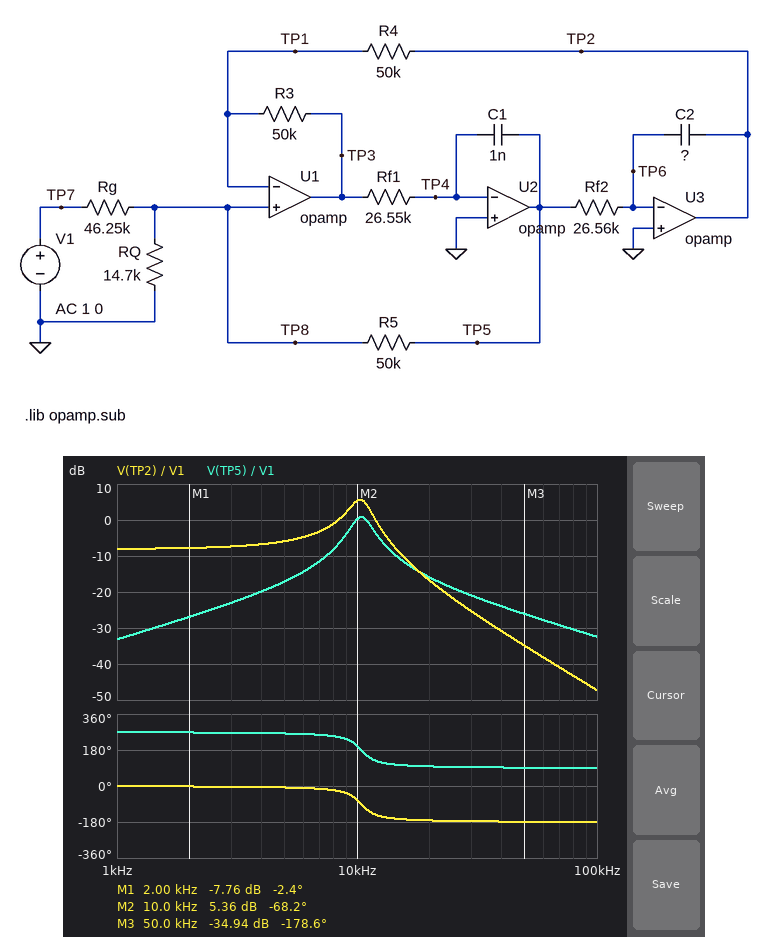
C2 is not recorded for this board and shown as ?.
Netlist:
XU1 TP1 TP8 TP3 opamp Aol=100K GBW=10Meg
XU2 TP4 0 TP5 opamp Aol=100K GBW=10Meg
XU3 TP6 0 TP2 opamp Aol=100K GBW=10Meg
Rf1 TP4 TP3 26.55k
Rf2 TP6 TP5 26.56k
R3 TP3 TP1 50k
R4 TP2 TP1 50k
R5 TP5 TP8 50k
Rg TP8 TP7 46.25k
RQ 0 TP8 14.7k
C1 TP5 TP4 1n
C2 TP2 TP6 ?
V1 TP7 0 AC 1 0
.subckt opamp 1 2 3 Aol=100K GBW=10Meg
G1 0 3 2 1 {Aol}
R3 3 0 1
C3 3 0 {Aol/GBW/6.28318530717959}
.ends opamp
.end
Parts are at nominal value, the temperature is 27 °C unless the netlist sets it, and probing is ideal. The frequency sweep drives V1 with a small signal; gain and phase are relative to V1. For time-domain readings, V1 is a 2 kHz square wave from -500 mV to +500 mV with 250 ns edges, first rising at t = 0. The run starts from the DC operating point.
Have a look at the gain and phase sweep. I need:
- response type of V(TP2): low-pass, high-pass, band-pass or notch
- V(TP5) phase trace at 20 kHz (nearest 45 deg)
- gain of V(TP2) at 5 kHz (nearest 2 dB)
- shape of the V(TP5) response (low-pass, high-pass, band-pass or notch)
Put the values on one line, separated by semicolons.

low-pass; 90 deg; -6 dB; band-pass
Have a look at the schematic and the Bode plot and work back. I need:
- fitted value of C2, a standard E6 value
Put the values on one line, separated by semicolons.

330 pF
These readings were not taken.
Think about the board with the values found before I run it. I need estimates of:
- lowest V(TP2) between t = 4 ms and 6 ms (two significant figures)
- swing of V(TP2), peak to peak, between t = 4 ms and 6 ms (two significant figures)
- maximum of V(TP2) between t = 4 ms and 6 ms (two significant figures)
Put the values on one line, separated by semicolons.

-540 mV; 1.1 V; 540 mV
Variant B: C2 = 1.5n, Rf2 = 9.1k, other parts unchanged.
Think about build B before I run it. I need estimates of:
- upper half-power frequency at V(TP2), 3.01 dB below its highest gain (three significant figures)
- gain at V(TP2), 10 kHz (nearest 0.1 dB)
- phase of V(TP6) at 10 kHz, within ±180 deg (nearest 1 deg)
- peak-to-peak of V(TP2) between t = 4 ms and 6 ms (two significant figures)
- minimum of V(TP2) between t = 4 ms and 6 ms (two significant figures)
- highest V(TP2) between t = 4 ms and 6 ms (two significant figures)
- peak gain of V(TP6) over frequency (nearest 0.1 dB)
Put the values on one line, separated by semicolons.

9.24 kHz; -2.6 dB; 125 deg; 840 mV; -420 mV; 420 mV; -57.9 dB
